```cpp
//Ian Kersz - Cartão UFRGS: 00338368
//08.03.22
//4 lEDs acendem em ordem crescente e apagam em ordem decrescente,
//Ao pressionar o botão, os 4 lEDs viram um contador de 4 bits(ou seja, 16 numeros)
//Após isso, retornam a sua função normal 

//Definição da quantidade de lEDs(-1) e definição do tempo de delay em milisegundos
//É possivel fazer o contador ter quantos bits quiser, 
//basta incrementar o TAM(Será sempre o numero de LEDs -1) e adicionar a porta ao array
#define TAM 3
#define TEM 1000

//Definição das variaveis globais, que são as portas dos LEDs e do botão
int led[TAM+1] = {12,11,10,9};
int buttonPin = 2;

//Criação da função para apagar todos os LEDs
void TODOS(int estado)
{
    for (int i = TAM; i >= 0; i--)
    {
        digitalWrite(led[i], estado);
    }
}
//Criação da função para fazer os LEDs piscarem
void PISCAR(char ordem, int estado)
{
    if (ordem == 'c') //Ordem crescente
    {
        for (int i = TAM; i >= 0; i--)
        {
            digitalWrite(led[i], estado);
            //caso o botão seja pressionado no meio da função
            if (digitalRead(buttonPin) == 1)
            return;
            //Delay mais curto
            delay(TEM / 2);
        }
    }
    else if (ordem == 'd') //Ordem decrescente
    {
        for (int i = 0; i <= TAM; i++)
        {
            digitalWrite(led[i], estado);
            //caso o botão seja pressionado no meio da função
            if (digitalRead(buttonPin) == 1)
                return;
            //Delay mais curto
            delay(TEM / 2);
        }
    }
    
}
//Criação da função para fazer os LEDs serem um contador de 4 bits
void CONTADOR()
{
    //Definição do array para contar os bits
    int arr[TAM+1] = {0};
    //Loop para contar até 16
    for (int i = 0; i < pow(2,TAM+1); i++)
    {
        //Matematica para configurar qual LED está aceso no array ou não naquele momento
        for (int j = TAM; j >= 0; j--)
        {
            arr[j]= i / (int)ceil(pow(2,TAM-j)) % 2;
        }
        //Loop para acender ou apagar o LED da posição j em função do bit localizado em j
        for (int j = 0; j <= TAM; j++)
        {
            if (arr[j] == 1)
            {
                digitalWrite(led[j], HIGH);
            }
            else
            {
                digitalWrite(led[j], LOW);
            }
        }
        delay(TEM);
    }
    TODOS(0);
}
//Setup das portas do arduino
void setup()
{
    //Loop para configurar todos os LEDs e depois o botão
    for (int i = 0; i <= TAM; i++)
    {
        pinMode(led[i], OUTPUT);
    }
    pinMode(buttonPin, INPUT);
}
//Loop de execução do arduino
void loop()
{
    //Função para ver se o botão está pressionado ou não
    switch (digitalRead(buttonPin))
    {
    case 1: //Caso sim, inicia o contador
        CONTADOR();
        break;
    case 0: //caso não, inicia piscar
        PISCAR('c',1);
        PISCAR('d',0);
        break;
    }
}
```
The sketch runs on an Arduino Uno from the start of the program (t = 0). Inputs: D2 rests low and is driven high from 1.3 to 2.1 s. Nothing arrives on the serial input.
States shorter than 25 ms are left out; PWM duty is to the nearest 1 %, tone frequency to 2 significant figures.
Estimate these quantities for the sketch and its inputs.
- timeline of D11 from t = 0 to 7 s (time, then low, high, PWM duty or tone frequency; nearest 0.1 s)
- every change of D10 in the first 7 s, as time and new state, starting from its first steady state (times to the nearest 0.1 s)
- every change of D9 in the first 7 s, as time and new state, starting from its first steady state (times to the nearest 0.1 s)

0 s low; 1 s high; 1.5 s low; 5.5 s high
0 s low; 0.5 s high; 1.5 s low; 3.5 s high; 5.5 s low
0 s high; 1.5 s low; 2.5 s high; 3.5 s low; 4.5 s high; 5.5 s low; 6.5 s high
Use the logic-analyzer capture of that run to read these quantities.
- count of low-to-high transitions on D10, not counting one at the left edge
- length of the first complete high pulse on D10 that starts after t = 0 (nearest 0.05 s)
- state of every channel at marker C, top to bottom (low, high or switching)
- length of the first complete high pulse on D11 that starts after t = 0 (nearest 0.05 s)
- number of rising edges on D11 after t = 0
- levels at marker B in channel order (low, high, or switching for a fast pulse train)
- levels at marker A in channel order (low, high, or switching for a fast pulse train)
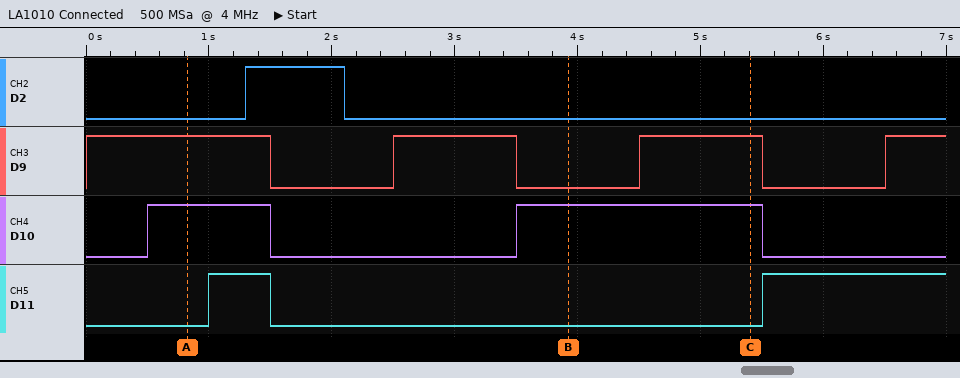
2
1.00 s
D2 low, D9 high, D10 high, D11 low
0.50 s
2
D2 low, D9 low, D10 high, D11 low
D2 low, D9 high, D10 high, D11 low
